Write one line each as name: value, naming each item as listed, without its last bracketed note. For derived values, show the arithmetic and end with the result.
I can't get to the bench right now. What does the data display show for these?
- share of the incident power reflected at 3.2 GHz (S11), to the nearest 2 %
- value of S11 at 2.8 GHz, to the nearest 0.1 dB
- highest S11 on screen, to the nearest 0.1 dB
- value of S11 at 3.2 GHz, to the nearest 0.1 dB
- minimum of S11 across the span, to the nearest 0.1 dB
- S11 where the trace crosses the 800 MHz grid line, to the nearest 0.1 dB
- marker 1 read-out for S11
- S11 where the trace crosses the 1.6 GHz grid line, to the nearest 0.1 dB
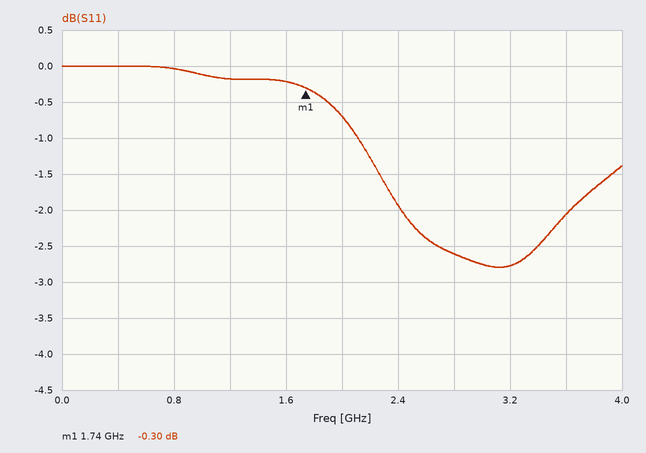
share of the incident power reflected at 3.2 GHz (S11), to the nearest 2 %: 10^(-2.8/10) ≈ 52 %
value of S11 at 2.8 GHz, to the nearest 0.1 dB: -2.6 dB
highest S11 on screen, to the nearest 0.1 dB: 0.0 dB
value of S11 at 3.2 GHz, to the nearest 0.1 dB: -2.8 dB
minimum of S11 across the span, to the nearest 0.1 dB: -2.8 dB
S11 where the trace crosses the 800 MHz grid line, to the nearest 0.1 dB: 0.0 dB
marker 1 read-out for S11: -0.30 dB
S11 where the trace crosses the 1.6 GHz grid line, to the nearest 0.1 dB: -0.2 dB
